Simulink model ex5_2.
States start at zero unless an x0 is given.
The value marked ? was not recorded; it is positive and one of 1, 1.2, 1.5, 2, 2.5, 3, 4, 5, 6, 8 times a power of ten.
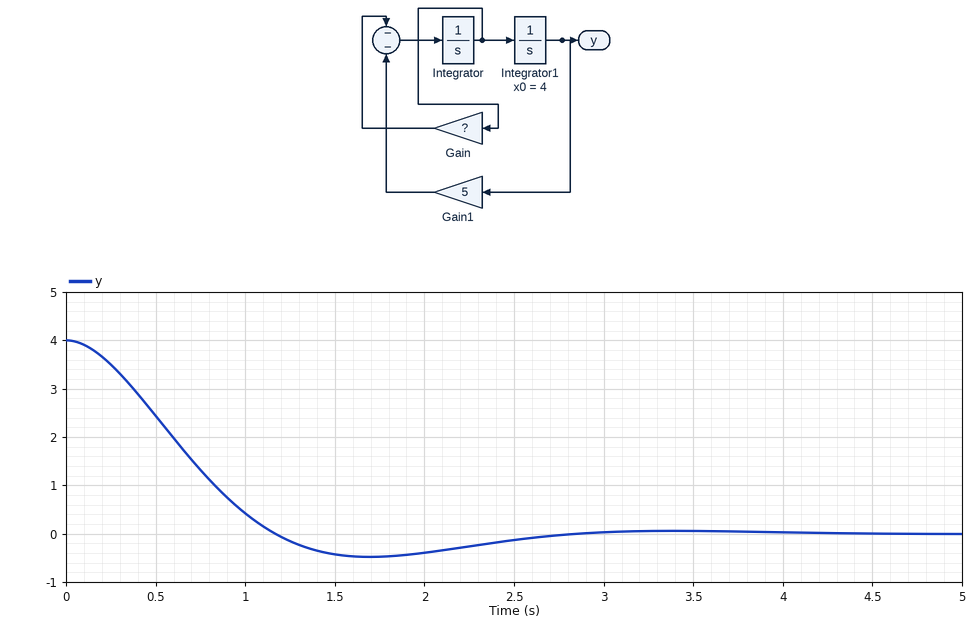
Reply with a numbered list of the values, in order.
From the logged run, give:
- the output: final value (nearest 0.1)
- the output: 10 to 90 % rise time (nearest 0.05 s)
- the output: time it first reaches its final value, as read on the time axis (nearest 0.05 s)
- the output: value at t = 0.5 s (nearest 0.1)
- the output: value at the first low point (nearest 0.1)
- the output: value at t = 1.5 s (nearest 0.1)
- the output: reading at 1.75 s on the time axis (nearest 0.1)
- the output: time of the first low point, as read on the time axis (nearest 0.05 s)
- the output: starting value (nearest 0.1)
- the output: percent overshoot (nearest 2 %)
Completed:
1. 0.0
2. 0.80 s
3. 1.15 s
4. 2.4
5. -0.5
6. -0.4
7. -0.5
8. 1.70 s
9. 4.0
10. 12 %
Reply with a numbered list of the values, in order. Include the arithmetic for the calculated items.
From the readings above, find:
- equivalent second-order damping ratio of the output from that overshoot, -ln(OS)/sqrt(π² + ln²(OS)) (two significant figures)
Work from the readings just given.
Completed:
1. ln(0.12) = -2.120; 2.120 / sqrt(9.870 + 4.496) = 0.56
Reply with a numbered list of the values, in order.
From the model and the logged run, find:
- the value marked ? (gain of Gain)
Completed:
1. 2.5
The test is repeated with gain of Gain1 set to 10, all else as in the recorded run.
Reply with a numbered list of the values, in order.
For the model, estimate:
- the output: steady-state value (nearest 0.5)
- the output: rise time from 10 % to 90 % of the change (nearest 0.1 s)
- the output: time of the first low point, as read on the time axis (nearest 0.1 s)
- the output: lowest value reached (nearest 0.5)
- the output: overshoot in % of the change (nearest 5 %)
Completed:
1. 0.0
2. 0.5 s
3. 1.1 s
4. -1.0
5. 25 %
